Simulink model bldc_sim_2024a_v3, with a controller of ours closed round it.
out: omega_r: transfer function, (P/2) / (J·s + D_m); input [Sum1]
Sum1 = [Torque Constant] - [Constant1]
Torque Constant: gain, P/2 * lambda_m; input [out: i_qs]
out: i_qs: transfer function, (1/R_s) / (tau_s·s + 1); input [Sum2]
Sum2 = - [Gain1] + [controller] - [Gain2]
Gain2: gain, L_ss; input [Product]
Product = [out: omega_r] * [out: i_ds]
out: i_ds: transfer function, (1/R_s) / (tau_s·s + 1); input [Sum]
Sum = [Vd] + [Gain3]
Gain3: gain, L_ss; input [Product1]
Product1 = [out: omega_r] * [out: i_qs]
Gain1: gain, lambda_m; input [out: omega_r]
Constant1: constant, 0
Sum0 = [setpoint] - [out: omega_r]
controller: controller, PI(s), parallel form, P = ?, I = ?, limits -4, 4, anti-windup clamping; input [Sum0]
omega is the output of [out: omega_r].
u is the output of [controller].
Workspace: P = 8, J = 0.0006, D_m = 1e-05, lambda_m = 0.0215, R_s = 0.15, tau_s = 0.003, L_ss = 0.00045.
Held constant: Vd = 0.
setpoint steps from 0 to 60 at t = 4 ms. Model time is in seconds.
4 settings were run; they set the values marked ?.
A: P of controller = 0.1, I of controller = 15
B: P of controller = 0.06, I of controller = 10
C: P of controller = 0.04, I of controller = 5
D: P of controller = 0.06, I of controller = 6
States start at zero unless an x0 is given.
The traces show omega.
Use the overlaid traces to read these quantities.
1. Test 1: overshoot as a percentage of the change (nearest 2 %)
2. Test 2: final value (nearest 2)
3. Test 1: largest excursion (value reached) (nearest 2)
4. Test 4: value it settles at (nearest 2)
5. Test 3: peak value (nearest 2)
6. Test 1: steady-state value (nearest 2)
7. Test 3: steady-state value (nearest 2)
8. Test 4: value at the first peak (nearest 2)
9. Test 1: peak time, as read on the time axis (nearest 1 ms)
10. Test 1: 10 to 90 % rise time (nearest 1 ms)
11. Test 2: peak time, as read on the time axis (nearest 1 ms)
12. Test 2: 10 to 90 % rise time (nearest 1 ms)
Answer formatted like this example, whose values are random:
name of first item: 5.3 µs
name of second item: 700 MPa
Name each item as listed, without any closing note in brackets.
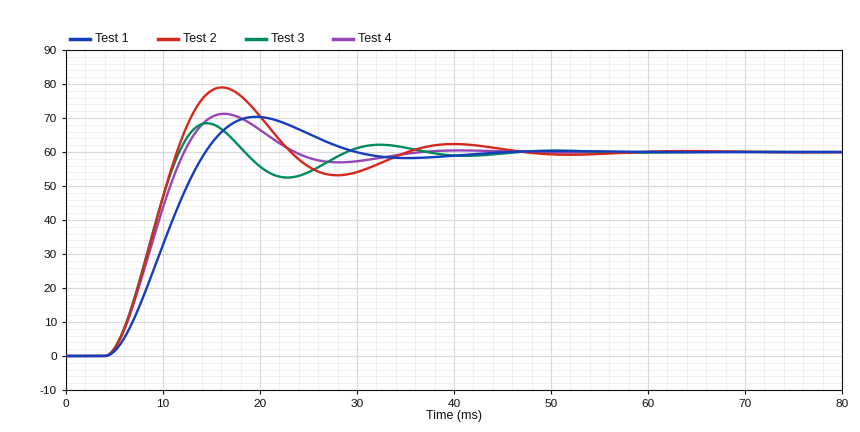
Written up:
Test 1: overshoot as a percentage of the change: 18 %
Test 2: final value: 60
Test 1: largest excursion (value reached): 70
Test 4: value it settles at: 60
Test 3: peak value: 68
Test 1: steady-state value: 60
Test 3: steady-state value: 60
Test 4: value at the first peak: 72
Test 1: peak time, as read on the time axis: 20 ms
Test 1: 10 to 90 % rise time: 7 ms
Test 2: peak time, as read on the time axis: 16 ms
Test 2: 10 to 90 % rise time: 5 ms
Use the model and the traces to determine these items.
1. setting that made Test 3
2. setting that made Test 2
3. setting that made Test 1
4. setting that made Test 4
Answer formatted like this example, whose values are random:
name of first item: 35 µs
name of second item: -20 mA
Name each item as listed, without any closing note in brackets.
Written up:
setting that made Test 3: A
setting that made Test 2: B
setting that made Test 1: C
setting that made Test 4: D
